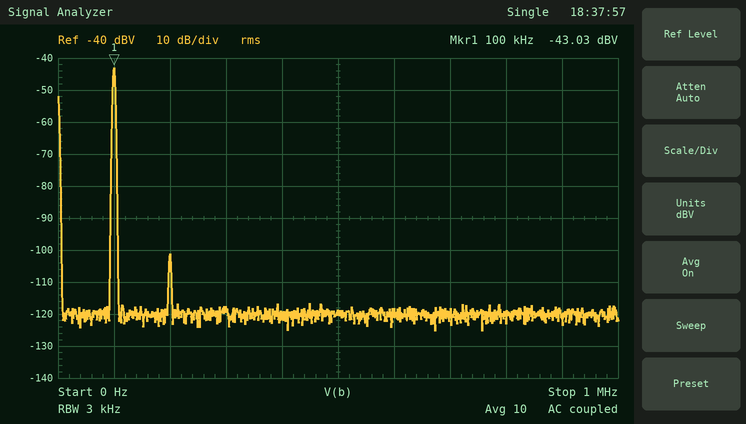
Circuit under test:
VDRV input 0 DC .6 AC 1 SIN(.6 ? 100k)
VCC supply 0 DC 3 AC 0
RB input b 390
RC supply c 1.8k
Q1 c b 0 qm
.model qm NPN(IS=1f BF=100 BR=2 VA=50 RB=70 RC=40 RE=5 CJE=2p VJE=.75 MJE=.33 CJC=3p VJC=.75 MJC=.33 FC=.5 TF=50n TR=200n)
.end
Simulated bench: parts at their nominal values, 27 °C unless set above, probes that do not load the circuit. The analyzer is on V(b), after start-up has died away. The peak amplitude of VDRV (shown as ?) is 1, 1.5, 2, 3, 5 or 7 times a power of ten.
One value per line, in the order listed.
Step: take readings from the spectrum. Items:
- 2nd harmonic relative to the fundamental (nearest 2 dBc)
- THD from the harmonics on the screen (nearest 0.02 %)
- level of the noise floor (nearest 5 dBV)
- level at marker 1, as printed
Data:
-58 dBc
0.12 %
-120 dBV
-43.03 dBV
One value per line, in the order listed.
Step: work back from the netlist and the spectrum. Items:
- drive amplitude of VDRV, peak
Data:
10 mV
